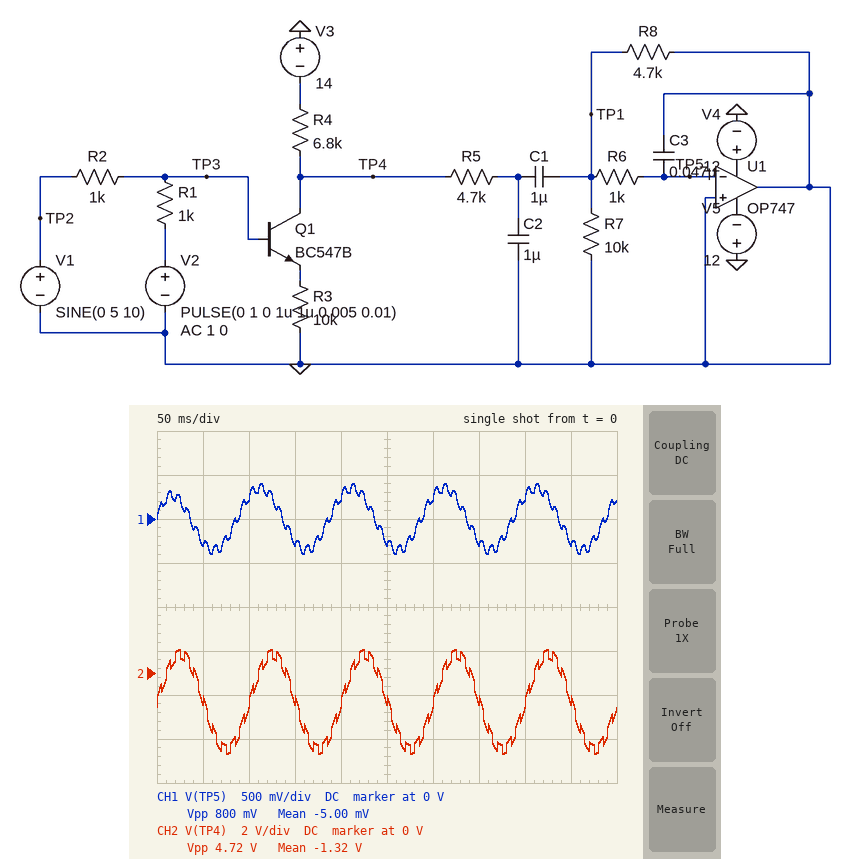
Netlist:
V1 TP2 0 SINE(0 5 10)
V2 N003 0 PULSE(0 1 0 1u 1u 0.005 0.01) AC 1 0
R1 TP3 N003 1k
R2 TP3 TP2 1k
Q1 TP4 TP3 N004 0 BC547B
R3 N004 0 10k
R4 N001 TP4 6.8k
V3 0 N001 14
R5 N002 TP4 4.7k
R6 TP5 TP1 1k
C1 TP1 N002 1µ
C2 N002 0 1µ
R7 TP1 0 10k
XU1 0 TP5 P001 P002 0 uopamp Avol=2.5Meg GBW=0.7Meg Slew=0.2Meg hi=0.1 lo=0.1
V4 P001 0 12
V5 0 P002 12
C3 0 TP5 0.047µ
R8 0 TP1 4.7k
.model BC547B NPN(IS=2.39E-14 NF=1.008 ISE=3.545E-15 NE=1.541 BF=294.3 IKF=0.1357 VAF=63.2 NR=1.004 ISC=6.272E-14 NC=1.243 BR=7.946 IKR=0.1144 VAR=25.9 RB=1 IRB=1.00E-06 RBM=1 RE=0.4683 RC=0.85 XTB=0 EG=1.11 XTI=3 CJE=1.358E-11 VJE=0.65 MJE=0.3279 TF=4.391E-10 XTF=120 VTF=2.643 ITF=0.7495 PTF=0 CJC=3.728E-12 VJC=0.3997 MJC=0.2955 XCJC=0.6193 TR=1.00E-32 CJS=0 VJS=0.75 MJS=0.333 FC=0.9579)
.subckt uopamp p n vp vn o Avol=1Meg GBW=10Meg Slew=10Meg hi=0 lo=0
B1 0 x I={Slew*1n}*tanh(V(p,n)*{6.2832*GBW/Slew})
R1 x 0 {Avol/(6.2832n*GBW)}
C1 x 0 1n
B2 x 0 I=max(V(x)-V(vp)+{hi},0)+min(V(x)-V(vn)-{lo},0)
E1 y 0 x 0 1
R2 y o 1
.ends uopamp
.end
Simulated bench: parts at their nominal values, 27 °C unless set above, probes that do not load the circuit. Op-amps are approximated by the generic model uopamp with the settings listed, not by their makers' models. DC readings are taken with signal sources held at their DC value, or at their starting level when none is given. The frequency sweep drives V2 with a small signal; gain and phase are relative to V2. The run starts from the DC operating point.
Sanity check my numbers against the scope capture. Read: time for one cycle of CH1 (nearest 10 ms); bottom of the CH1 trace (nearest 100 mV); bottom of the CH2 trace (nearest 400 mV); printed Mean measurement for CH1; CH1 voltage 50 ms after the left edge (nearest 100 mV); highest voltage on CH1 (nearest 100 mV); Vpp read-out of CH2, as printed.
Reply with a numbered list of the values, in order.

1. 100 ms
2. -400 mV
3. -3.6 V
4. -5.00 mV
5. -300 mV
6. 400 mV
7. 4.72 V
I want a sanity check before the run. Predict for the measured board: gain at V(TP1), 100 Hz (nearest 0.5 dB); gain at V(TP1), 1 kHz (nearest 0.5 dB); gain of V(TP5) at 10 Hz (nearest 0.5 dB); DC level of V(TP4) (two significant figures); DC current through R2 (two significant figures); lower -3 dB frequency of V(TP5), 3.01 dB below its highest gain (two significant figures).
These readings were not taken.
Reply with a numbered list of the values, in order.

1. -21.5 dB
2. -38.0 dB
3. -23.0 dB
4. -1.5 V
5. 840 µA
6. 11 Hz
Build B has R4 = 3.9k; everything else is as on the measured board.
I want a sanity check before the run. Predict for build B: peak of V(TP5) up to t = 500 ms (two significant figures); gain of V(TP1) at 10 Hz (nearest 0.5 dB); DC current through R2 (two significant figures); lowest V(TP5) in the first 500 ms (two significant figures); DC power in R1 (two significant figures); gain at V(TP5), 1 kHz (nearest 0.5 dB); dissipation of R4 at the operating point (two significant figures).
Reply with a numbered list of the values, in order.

1. 380 mV
2. -23.5 dB
3. 1.4 mA
4. -380 mV
5. 2.0 mW
6. -39.0 dB
7. 36 mW
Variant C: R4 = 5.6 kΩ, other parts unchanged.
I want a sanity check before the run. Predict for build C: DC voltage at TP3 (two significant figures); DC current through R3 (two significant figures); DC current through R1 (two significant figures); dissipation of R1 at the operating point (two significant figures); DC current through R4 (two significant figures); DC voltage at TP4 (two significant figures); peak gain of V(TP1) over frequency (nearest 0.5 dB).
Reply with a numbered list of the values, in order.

1. -1.0 V
2. 170 µA
3. 1.0 mA
4. 1.0 mW
5. 2.2 mA
6. -1.7 V
7. -20.0 dB
